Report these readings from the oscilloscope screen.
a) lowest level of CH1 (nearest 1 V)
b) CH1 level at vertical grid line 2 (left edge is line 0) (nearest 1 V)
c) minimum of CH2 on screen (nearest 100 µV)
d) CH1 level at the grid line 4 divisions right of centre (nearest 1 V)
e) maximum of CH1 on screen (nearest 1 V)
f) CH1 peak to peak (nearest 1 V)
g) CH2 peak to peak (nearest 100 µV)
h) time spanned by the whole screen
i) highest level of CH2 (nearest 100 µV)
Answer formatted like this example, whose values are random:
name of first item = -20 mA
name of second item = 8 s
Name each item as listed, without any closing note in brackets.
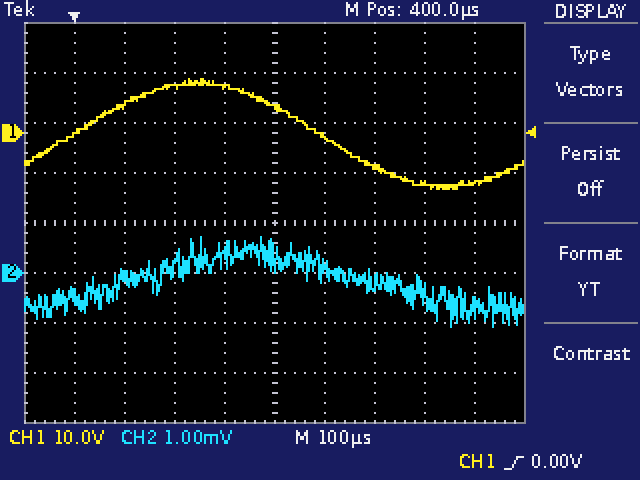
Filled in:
lowest level of CH1 = -11 V
CH1 level at vertical grid line 2 (left edge is line 0) = 6 V
minimum of CH2 on screen = -1.1 mV
CH1 level at the grid line 4 divisions right of centre = -10 V
maximum of CH1 on screen = 11 V
CH1 peak to peak = 22 V
CH2 peak to peak = 1.8 mV
time spanned by the whole screen = 1 ms
highest level of CH2 = 700 µV
